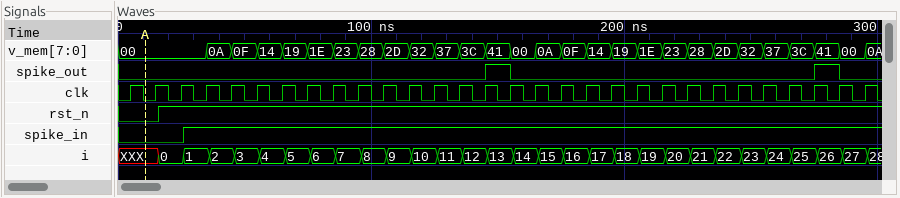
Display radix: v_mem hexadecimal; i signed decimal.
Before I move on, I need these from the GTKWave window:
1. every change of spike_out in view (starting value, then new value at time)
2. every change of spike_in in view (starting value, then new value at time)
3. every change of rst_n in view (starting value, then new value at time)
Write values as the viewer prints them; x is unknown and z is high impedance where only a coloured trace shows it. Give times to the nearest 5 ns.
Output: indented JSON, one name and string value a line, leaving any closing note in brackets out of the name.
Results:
{
  "every change of spike_out in view": "0, 1 at 145 ns, 0 at 155 ns, 1 at 275 ns, 0 at 285 ns",
  "every change of spike_in in view": "0, 1 at 25 ns",
  "every change of rst_n in view": "0, 1 at 15 ns"
}
